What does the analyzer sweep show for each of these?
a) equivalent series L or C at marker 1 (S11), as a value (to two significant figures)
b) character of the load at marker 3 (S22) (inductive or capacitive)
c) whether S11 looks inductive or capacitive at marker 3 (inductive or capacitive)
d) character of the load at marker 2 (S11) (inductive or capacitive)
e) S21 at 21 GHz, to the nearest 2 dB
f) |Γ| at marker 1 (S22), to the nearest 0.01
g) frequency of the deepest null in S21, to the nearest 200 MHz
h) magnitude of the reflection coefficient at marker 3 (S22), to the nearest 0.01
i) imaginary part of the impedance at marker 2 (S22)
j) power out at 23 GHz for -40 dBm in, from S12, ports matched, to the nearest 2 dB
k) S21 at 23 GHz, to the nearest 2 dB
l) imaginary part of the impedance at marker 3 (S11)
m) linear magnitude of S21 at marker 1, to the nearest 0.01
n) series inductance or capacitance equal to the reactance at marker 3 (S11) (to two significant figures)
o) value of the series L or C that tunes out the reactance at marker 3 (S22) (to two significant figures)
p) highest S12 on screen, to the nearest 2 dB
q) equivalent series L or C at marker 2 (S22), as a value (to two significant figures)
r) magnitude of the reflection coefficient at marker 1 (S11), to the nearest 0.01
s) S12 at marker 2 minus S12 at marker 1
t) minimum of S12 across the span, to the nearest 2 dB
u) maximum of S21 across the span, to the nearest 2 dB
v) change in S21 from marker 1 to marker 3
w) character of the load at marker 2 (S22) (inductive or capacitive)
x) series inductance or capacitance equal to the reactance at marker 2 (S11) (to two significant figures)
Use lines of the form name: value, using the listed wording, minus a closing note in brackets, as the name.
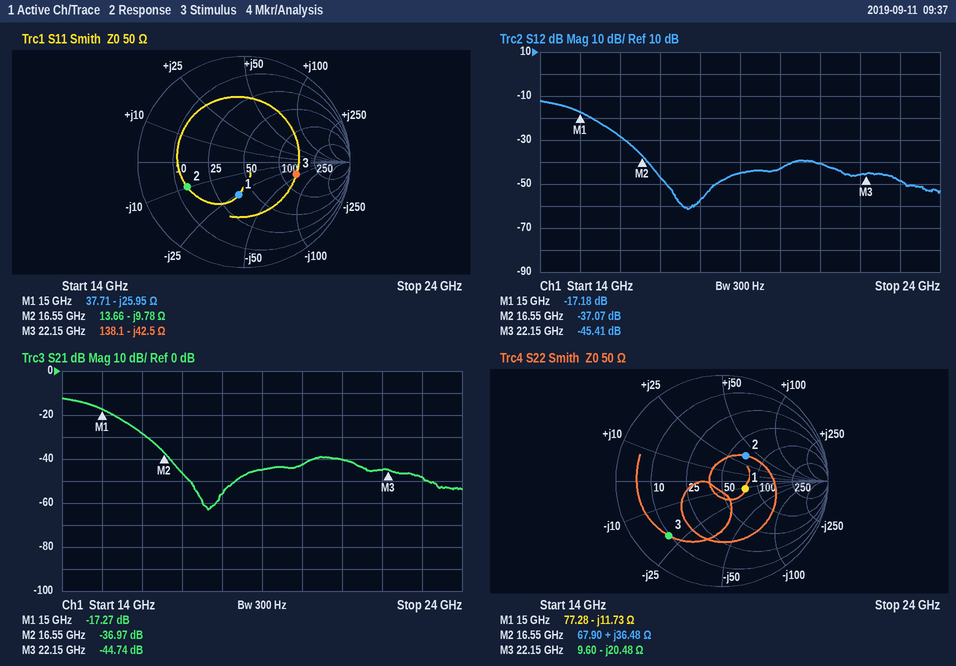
equivalent series L or C at marker 1 (S11), as a value: 410 fF
character of the load at marker 3 (S22): capacitive
whether S11 looks inductive or capacitive at marker 3: capacitive
character of the load at marker 2 (S11): capacitive
S21 at 21 GHz, to the nearest 2 dB: -40 dB
|Γ| at marker 1 (S22), to the nearest 0.01: 0.23
frequency of the deepest null in S21, to the nearest 200 MHz: 17.6 GHz
magnitude of the reflection coefficient at marker 3 (S22), to the nearest 0.01: 0.72
imaginary part of the impedance at marker 2: +36.48 Ω
power out at 23 GHz for -40 dBm in, from S12, ports matched, to the nearest 2 dB: -88 dBm
S21 at 23 GHz, to the nearest 2 dB: -48 dB
imaginary part of the impedance at marker 3: -42.5 Ω
linear magnitude of S21 at marker 1, to the nearest 0.01: 0.14
series inductance or capacitance equal to the reactance at marker 3 (S11): 170 fF
value of the series L or C that tunes out the reactance at marker 3 (S22): 150 pH
highest S12 on screen, to the nearest 2 dB: -12 dB
equivalent series L or C at marker 2 (S22), as a value: 350 pH
magnitude of the reflection coefficient at marker 1 (S11), to the nearest 0.01: 0.31
S12 at marker 2 minus S12 at marker 1: -19.89 dB
minimum of S12 across the span, to the nearest 2 dB: -62 dB
maximum of S21 across the span, to the nearest 2 dB: -12 dB
change in S21 from marker 1 to marker 3: -27.47 dB
character of the load at marker 2 (S22): inductive
series inductance or capacitance equal to the reactance at marker 2 (S11): 980 fF
